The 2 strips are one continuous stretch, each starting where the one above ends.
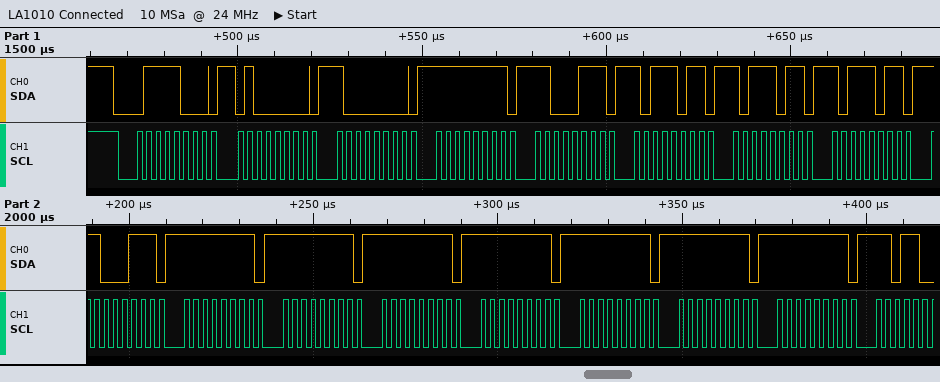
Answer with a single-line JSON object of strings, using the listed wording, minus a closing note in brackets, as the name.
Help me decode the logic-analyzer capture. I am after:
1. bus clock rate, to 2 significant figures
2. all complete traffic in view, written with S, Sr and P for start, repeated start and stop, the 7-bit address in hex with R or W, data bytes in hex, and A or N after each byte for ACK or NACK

{"bus clock rate, to 2 significant figures": "400 kHz", "all complete traffic in view, written with S, Sr and P for start, repeated start and stop, the 7-bit address in hex with R or W, data bytes in hex, and A or N after each byte for ACK or NACK": "S 3CW A 40 A 80 A FF A C7 A BB A BB A BB A C7 A FF A FF A FF A FF A FF A FF A FF A"}
